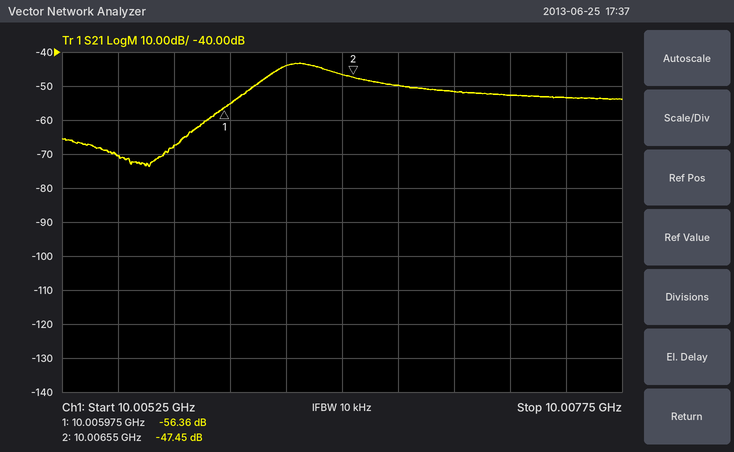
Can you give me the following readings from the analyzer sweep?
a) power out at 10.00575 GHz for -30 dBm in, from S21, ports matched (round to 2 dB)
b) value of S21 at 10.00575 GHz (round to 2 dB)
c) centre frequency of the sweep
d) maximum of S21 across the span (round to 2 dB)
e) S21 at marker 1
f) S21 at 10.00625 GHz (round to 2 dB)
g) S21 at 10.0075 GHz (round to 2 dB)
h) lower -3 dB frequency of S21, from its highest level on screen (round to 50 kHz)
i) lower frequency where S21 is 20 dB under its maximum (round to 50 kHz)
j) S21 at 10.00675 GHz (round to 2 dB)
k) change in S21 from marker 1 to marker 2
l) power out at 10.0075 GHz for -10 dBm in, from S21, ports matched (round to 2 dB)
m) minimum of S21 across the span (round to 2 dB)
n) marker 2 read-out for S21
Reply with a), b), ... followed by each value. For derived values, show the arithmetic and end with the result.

a) -30 dBm + (-68 dB) = -98 dBm
b) -68 dB
c) 10.0065 GHz
d) -44 dB
e) -56.36 dB
f) -44 dB
g) -54 dB
h) 10.00620 GHz
i) 10.00585 GHz
j) -50 dB
k) -47.45 − (-56.36) = 8.91 dB
l) -10 dBm + (-54 dB) = -64 dBm
m) -74 dB
n) -47.45 dB
